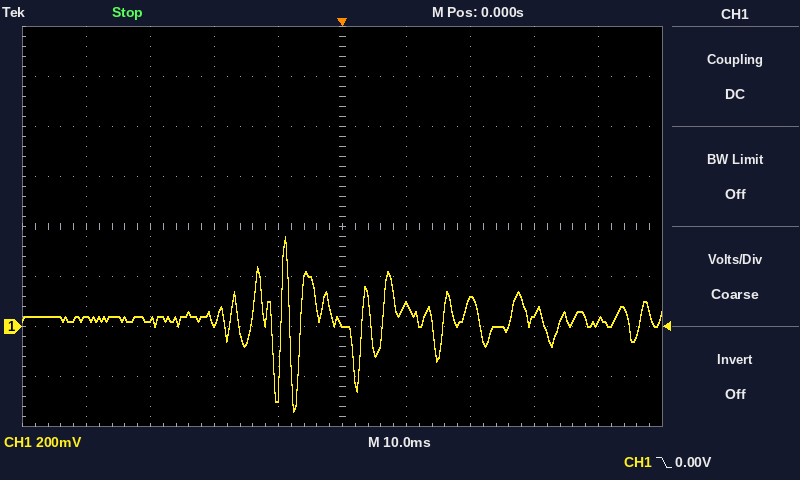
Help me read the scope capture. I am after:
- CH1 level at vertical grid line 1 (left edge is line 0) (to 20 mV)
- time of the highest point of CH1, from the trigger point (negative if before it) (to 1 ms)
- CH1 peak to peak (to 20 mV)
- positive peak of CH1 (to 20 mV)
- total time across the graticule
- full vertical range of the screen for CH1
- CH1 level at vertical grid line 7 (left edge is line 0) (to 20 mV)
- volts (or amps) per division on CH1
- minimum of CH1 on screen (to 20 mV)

40 mV
-9 ms
700 mV
360 mV
100 ms
1.6 V
100 mV
200 mV
-340 mV
